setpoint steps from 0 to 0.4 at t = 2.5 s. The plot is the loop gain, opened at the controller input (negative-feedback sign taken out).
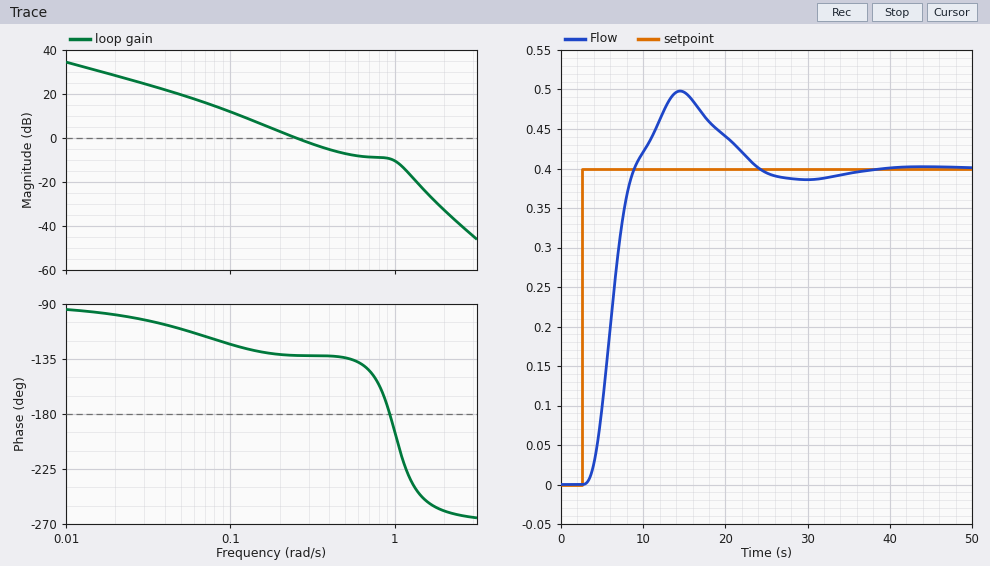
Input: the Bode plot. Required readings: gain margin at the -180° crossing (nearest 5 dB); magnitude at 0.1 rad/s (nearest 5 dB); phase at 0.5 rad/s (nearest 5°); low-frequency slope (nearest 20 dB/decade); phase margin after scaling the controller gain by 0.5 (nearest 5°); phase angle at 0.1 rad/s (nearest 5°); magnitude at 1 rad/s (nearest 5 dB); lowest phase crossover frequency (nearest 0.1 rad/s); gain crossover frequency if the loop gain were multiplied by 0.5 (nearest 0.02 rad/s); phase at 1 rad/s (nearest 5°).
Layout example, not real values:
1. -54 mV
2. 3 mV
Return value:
1. 10 dB
2. 10 dB
3. -135°
4. -20 dB/decade
5. 50°
6. -125°
7. -10 dB
8. 0.9 rad/s
9. 0.16 rad/s
10. -195°
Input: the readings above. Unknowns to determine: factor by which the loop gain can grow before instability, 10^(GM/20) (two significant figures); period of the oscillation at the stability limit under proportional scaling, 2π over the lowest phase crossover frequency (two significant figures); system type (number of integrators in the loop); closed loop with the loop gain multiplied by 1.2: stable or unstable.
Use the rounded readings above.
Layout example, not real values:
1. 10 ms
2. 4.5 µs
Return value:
1. 3.2
2. 7.0 s
3. 1
4. stable
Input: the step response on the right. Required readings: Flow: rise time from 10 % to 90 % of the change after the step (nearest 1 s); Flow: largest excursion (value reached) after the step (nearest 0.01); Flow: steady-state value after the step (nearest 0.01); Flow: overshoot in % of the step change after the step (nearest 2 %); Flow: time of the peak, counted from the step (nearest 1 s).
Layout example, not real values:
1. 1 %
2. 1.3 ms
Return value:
1. 4 s
2. 0.50
3. 0.40
4. 24 %
5. 12 s
